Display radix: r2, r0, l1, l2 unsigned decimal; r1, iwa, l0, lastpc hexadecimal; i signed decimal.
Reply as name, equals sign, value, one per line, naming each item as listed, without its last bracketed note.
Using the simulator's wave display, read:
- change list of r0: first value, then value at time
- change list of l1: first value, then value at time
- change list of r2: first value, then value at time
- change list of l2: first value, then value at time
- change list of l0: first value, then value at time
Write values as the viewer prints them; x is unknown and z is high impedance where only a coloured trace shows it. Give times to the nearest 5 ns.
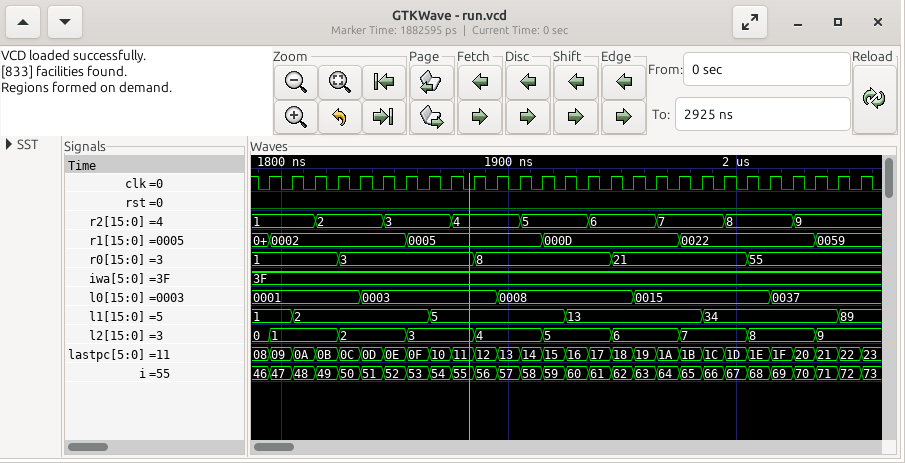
change list of r0: first value, then value at time = 1, 3 at 1825 ns, 8 at 1885 ns, 21 at 1945 ns, 55 at 2005 ns
change list of l1: first value, then value at time = 1, 2 at 1805 ns, 5 at 1865 ns, 13 at 1925 ns, 34 at 1985 ns, 89 at 2045 ns
change list of r2: first value, then value at time = 1, 2 at 1815 ns, 3 at 1845 ns, 4 at 1875 ns, 5 at 1905 ns, 6 at 1935 ns, 7 at 1965 ns, 8 at 1995 ns, 9 at 2025 ns
change list of l2: first value, then value at time = 0, 1 at 1795 ns, 2 at 1825 ns, 3 at 1855 ns, 4 at 1885 ns, 5 at 1915 ns, 6 at 1945 ns, 7 at 1975 ns, 8 at 2005 ns, 9 at 2035 ns
change list of l0: first value, then value at time = 0001, 0003 at 1835 ns, 0008 at 1895 ns, 0015 at 1955 ns, 0037 at 2015 ns
